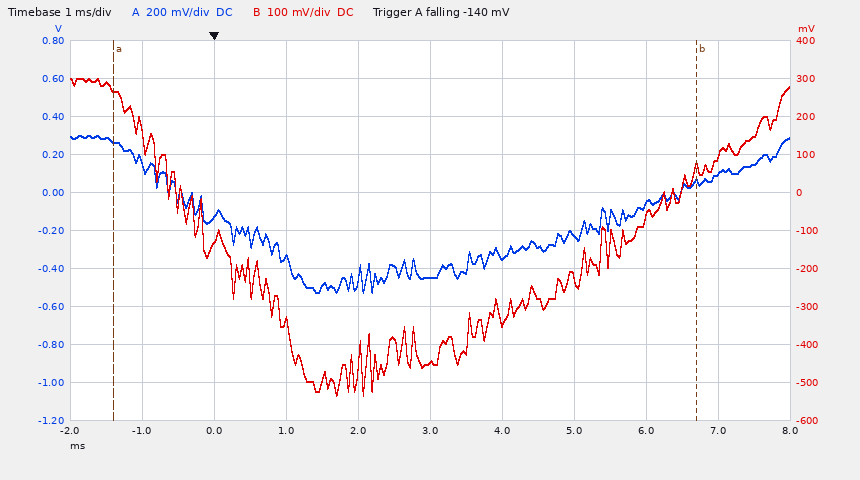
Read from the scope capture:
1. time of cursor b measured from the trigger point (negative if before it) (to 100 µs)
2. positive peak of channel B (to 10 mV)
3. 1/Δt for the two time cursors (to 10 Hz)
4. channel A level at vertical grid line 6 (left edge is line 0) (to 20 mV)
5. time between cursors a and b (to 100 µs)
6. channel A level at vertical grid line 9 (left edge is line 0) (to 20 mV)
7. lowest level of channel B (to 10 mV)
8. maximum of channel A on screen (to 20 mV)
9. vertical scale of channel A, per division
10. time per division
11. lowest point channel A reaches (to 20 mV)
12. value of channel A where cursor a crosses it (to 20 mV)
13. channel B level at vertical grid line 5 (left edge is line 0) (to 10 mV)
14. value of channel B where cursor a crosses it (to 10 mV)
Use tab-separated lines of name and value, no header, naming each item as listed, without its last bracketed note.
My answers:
time of cursor b measured from the trigger point (negative if before it)	+6.7 ms
positive peak of channel B	300 mV
1/Δt for the two time cursors	120 Hz
channel A level at vertical grid line 6 (left edge is line 0)	-340 mV
time between cursors a and b	8.1 ms
channel A level at vertical grid line 9 (left edge is line 0)	100 mV
lowest level of channel B	-530 mV
maximum of channel A on screen	300 mV
vertical scale of channel A, per division	200 mV
time per division	1 ms
lowest point channel A reaches	-520 mV
value of channel A where cursor a crosses it	280 mV
channel B level at vertical grid line 5 (left edge is line 0)	-450 mV
value of channel B where cursor a crosses it	270 mV
